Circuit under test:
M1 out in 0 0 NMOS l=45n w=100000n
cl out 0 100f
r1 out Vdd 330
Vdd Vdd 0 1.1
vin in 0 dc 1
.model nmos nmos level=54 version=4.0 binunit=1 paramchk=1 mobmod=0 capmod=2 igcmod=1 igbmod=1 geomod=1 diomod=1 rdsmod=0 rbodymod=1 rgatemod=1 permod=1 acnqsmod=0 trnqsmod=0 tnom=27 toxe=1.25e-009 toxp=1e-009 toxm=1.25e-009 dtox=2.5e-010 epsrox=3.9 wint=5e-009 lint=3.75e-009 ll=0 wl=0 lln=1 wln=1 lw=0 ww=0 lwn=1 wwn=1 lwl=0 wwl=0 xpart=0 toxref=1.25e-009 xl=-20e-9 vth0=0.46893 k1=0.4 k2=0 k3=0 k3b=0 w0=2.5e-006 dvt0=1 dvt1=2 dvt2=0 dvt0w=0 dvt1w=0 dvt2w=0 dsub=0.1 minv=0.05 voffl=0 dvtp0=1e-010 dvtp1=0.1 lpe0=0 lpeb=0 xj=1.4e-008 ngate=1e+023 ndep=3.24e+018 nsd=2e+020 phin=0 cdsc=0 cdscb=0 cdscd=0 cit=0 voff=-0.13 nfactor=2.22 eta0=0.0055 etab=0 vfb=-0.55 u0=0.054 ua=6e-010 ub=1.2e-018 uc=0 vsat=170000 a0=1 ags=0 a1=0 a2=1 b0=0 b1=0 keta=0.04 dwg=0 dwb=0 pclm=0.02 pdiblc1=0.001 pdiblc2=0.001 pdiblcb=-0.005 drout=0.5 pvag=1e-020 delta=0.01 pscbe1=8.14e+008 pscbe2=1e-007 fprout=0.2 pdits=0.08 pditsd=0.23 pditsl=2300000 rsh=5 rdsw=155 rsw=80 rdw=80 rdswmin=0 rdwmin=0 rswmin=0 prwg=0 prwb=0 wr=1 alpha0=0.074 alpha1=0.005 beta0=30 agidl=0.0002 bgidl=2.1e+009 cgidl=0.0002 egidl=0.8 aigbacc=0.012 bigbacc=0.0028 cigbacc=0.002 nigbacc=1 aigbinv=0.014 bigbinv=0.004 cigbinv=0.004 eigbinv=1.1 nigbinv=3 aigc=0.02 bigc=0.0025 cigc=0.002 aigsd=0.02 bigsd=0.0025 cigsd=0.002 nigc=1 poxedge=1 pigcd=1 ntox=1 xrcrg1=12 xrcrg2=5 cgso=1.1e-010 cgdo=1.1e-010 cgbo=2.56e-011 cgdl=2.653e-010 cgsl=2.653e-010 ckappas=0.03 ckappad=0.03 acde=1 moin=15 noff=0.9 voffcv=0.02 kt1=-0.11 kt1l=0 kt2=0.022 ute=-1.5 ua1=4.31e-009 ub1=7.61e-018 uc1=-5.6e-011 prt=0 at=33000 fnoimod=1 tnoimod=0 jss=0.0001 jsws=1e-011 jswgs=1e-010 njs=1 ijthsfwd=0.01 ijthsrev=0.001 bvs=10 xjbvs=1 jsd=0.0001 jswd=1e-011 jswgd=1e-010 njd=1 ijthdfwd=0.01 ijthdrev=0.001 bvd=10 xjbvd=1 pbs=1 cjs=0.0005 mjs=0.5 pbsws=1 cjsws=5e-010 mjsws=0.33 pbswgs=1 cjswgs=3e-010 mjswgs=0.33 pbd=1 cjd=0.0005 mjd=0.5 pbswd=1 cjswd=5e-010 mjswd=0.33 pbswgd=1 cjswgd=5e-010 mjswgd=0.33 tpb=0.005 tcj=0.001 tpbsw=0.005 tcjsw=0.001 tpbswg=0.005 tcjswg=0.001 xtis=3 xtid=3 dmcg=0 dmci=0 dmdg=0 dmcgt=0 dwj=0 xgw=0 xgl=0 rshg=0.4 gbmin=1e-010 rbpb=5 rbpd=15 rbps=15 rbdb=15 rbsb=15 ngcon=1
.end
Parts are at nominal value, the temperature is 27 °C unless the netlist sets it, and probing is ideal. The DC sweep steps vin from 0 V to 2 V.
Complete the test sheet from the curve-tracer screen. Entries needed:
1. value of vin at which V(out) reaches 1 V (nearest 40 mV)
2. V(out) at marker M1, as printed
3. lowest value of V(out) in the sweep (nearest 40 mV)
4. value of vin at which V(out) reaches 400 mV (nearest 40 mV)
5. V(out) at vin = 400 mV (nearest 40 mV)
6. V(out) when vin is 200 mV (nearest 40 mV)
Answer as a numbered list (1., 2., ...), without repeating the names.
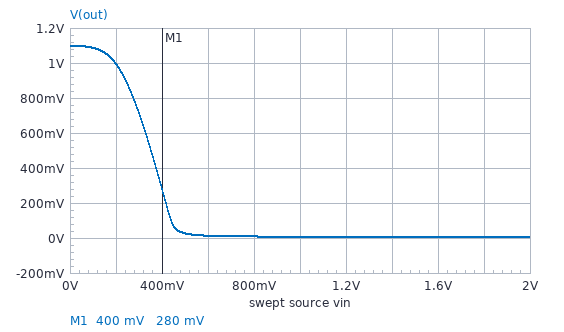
1. 200 mV
2. 280 mV
3. 0 V
4. 360 mV
5. 280 mV
6. 1.00 V
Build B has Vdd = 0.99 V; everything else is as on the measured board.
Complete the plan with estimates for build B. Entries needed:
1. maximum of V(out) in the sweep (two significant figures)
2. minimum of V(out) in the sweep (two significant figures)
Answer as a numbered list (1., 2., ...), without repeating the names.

1. 990 mV
2. 6.1 mV
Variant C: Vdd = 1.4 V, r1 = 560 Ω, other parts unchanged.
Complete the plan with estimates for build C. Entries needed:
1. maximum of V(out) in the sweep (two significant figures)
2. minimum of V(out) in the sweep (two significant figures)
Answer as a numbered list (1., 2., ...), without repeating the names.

1. 1.4 V
2. 5.1 mV
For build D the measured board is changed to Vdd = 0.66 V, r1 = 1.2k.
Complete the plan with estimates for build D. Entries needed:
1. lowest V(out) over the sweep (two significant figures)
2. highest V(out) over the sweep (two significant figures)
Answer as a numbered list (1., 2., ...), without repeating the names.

1. 1.1 mV
2. 660 mV
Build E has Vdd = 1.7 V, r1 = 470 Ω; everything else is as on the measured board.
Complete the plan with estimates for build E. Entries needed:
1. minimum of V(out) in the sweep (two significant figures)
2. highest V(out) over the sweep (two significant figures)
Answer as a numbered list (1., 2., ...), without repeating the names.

1. 7.4 mV
2. 1.6 V
